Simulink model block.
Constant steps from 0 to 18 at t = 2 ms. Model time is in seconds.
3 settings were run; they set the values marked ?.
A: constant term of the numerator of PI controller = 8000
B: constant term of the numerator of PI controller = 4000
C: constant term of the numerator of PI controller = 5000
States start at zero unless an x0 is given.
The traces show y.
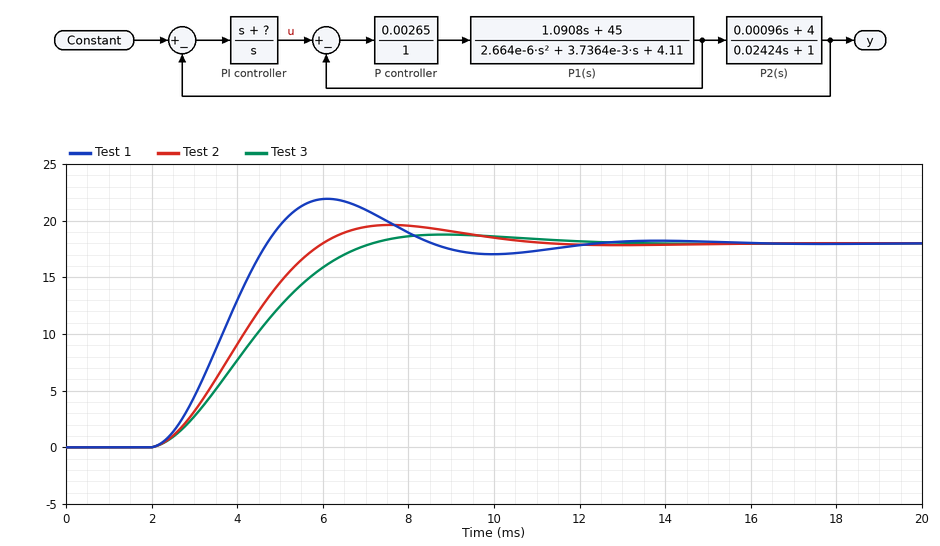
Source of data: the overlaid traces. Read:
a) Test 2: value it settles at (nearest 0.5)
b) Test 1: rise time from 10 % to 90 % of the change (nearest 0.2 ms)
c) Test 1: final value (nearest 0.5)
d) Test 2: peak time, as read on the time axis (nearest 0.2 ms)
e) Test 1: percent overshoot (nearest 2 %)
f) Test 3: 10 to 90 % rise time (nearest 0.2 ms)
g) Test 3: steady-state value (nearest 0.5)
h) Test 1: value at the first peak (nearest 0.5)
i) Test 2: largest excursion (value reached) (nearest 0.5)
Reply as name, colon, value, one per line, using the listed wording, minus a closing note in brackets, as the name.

Test 2: value it settles at: 18.0
Test 1: rise time from 10 % to 90 % of the change: 1.8 ms
Test 1: final value: 18.0
Test 2: peak time, as read on the time axis: 7.6 ms
Test 1: percent overshoot: 22 %
Test 3: 10 to 90 % rise time: 3.4 ms
Test 3: steady-state value: 18.0
Test 1: value at the first peak: 22.0
Test 2: largest excursion (value reached): 19.5
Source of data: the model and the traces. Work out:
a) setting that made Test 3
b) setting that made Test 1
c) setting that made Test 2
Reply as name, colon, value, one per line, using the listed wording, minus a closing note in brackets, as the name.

setting that made Test 3: B
setting that made Test 1: A
setting that made Test 2: C
